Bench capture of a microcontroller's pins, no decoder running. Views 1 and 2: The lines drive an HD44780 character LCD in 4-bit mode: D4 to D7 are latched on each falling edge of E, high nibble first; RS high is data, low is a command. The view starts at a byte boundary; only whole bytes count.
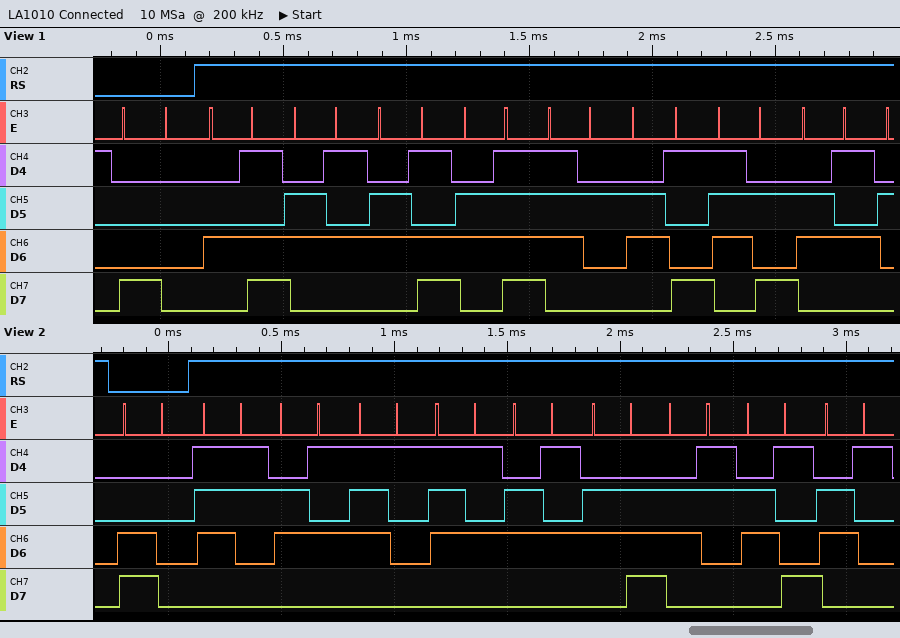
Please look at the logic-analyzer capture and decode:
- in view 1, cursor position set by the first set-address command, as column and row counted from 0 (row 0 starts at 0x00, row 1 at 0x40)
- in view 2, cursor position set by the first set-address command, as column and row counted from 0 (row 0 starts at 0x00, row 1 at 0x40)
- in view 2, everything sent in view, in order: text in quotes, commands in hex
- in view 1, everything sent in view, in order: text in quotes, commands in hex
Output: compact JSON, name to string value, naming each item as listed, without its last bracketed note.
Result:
{"in view 1, cursor position set by the first set-address command, as column and row counted from 0": "column 0, row 0", "in view 2, cursor position set by the first set-address command, as column and row counted from 0": "column 0, row 1", "in view 2, everything sent in view, in order: text in quotes, commands in hex": "0xC0 \"sequencia\"", "in view 1, everything sent in view, in order: text in quotes, commands in hex": "0x80 \"Memorize\""}
